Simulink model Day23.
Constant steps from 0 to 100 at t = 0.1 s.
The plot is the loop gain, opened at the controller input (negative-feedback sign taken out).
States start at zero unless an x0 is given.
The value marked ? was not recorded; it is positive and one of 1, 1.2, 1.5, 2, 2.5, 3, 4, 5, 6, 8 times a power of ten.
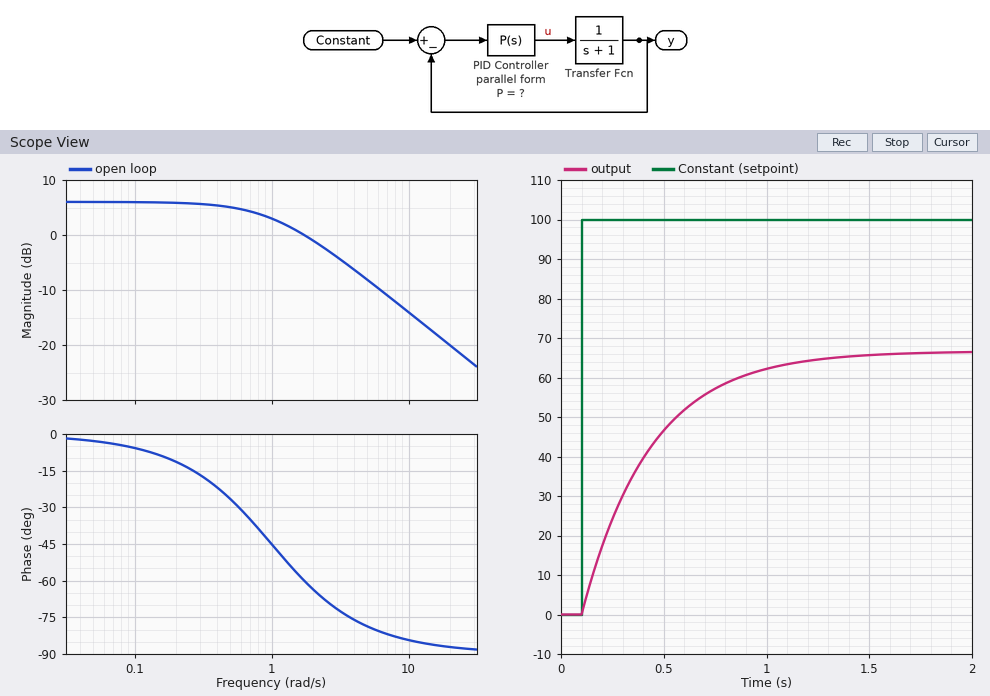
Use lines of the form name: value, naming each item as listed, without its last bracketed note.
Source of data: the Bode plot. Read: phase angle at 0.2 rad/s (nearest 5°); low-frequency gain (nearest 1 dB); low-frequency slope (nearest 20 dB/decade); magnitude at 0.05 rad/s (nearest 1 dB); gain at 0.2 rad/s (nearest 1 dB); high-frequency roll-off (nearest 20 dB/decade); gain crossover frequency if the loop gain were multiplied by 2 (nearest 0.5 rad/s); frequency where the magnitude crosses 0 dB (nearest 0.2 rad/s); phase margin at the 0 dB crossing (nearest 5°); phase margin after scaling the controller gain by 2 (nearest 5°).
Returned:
phase angle at 0.2 rad/s: -10°
low-frequency gain: 6 dB
low-frequency slope: 0 dB/decade
magnitude at 0.05 rad/s: 6 dB
gain at 0.2 rad/s: 6 dB
high-frequency roll-off: -20 dB/decade
gain crossover frequency if the loop gain were multiplied by 2: 4.0 rad/s
frequency where the magnitude crosses 0 dB: 1.8 rad/s
phase margin at the 0 dB crossing: 120°
phase margin after scaling the controller gain by 2: 105°
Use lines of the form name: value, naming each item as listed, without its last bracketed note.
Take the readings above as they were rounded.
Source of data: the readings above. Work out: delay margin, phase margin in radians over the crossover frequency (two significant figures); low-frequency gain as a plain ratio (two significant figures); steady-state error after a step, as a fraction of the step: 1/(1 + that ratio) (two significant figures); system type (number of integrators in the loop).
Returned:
delay margin, phase margin in radians over the crossover frequency: 1.2 s
low-frequency gain as a plain ratio: 2.0
steady-state error after a step, as a fraction of the step: 1/(1 + that ratio): 0.33
system type: 0
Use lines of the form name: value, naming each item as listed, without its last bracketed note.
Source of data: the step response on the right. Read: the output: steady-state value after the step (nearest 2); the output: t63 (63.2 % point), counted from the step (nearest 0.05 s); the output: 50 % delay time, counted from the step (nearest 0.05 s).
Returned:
the output: steady-state value after the step: 66
the output: t63 (63.2 % point), counted from the step: 0.35 s
the output: 50 % delay time, counted from the step: 0.25 s
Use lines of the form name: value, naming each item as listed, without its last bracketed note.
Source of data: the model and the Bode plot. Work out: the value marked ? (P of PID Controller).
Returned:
the value marked ?: 2
